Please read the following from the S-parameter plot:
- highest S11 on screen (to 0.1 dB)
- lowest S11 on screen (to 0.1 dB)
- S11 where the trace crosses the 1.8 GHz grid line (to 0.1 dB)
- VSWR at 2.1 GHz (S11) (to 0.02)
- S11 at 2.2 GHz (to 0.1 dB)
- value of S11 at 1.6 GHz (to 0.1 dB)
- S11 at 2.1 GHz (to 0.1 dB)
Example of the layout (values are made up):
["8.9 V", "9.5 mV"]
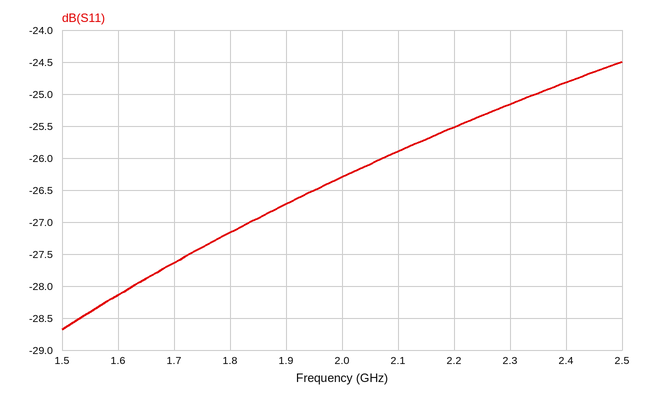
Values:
["-24.5 dB", "-28.7 dB", "-27.2 dB", "1.10", "-25.5 dB", "-28.1 dB", "-25.9 dB"]
